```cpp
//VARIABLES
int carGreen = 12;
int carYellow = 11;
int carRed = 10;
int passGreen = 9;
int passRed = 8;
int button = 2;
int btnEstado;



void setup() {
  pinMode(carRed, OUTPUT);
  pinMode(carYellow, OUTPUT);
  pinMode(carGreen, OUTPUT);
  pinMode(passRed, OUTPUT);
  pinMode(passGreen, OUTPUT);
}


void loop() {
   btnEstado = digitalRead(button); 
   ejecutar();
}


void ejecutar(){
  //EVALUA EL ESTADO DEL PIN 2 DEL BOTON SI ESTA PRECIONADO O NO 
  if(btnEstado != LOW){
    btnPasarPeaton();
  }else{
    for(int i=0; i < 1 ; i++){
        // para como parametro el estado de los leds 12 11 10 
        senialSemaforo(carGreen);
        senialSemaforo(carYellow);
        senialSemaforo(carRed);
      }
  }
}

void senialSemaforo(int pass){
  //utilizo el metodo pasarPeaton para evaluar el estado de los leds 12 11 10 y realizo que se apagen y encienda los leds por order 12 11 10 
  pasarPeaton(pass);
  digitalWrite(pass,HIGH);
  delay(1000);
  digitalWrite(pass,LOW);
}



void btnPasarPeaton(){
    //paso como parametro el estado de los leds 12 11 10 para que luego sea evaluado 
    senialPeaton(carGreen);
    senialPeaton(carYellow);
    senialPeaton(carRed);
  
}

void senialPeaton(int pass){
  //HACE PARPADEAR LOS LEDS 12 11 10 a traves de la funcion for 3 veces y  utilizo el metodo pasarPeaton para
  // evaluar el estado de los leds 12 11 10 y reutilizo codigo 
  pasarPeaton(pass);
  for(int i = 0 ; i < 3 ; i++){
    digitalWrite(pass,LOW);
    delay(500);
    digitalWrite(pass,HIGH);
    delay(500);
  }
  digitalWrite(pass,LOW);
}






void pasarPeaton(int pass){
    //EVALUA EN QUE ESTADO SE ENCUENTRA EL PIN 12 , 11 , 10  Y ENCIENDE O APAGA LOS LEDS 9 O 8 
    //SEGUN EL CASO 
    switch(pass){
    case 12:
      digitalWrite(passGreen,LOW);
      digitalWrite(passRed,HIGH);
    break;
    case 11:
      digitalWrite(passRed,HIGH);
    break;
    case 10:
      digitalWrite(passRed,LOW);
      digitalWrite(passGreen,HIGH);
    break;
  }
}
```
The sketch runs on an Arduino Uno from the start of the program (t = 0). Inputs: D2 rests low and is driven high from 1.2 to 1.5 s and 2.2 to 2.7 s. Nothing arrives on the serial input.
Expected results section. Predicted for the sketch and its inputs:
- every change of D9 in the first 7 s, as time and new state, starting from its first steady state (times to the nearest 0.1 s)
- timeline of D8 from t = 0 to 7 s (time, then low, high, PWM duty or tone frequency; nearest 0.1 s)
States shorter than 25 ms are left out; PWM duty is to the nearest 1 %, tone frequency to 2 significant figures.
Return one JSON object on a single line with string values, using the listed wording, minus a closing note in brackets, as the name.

{"every change of D9 in the first 7 s, as time and new state, starting from its first steady state": "0 s low; 2 s high; 3 s low; 5 s high; 6 s low", "timeline of D8 from t = 0 to 7 s": "0 s high; 2 s low; 3 s high; 5 s low; 6 s high"}
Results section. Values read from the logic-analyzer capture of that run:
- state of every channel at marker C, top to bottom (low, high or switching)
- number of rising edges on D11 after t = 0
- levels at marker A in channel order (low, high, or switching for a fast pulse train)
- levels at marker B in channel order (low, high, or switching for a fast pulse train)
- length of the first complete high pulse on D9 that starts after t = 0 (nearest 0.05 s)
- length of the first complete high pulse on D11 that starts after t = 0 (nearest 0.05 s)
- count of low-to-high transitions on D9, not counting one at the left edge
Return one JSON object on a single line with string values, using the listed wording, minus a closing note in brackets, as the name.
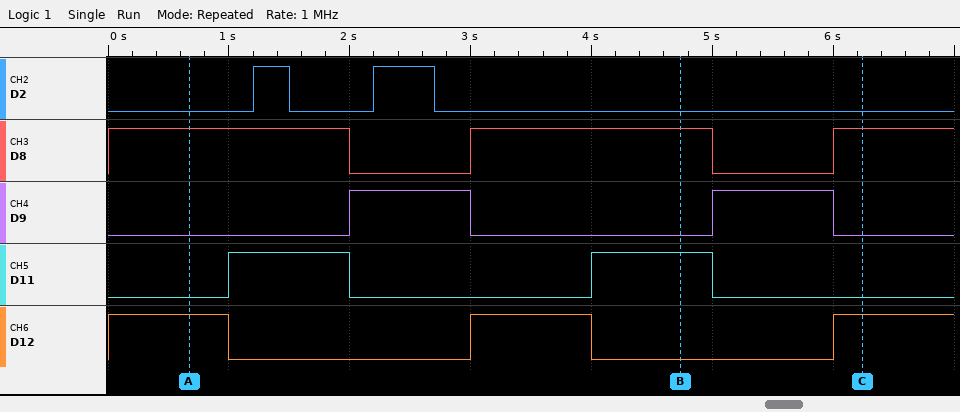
{"state of every channel at marker C, top to bottom": "D2 low, D8 high, D9 low, D11 low, D12 high", "number of rising edges on D11 after t = 0": "2", "levels at marker A in channel order": "D2 low, D8 high, D9 low, D11 low, D12 high", "levels at marker B in channel order": "D2 low, D8 high, D9 low, D11 high, D12 low", "length of the first complete high pulse on D9 that starts after t = 0": "1.00 s", "length of the first complete high pulse on D11 that starts after t = 0": "1.00 s", "count of low-to-high transitions on D9, not counting one at the left edge": "2"}
